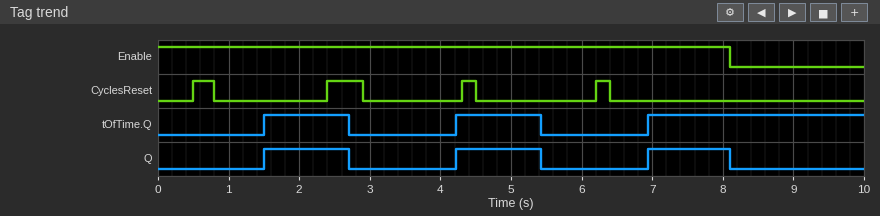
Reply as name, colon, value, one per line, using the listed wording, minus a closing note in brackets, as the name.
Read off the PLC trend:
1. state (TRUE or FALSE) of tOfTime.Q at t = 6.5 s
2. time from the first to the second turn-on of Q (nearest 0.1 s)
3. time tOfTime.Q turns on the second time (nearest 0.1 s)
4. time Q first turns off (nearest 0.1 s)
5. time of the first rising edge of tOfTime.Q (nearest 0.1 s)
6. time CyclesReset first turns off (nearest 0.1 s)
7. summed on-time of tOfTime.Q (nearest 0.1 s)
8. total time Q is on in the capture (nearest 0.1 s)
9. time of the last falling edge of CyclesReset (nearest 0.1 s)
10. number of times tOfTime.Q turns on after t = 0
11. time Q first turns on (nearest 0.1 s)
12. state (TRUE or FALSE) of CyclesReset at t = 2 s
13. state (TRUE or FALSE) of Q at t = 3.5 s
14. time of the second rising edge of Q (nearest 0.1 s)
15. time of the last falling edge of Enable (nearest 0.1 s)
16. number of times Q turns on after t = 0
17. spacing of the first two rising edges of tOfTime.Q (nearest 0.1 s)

state (TRUE or FALSE) of tOfTime.Q at t = 6.5 s: FALSE
time from the first to the second turn-on of Q: 2.7 s
time tOfTime.Q turns on the second time: 4.2 s
time Q first turns off: 2.7 s
time of the first rising edge of tOfTime.Q: 1.5 s
time CyclesReset first turns off: 0.8 s
summed on-time of tOfTime.Q: 5.5 s
total time Q is on in the capture: 3.6 s
time of the last falling edge of CyclesReset: 6.4 s
number of times tOfTime.Q turns on after t = 0: 3
time Q first turns on: 1.5 s
state (TRUE or FALSE) of CyclesReset at t = 2 s: FALSE
state (TRUE or FALSE) of Q at t = 3.5 s: FALSE
time of the second rising edge of Q: 4.2 s
time of the last falling edge of Enable: 8.1 s
number of times Q turns on after t = 0: 3
spacing of the first two rising edges of tOfTime.Q: 2.7 s
